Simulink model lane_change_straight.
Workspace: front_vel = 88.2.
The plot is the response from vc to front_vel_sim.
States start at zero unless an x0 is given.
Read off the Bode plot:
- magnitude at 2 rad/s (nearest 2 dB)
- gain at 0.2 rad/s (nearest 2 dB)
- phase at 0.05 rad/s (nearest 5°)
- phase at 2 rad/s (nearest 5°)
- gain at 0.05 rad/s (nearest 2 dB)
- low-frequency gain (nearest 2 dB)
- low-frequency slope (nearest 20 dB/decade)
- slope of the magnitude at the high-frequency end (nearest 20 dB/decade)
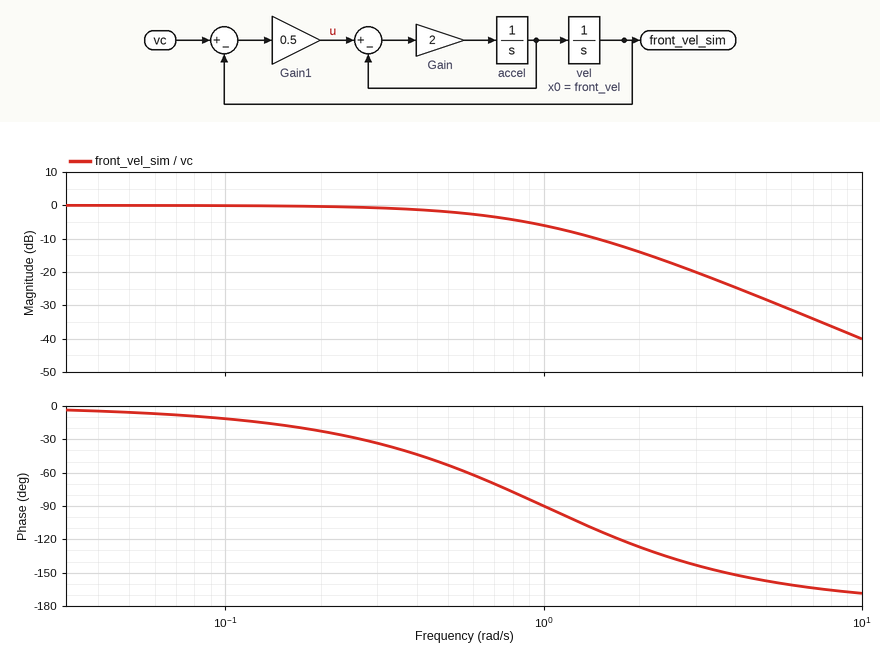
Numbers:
-14 dB
0 dB
-5°
-125°
0 dB
0 dB
0 dB/decade
-40 dB/decade
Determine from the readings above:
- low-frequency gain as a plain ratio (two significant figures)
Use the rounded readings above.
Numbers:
1.0
